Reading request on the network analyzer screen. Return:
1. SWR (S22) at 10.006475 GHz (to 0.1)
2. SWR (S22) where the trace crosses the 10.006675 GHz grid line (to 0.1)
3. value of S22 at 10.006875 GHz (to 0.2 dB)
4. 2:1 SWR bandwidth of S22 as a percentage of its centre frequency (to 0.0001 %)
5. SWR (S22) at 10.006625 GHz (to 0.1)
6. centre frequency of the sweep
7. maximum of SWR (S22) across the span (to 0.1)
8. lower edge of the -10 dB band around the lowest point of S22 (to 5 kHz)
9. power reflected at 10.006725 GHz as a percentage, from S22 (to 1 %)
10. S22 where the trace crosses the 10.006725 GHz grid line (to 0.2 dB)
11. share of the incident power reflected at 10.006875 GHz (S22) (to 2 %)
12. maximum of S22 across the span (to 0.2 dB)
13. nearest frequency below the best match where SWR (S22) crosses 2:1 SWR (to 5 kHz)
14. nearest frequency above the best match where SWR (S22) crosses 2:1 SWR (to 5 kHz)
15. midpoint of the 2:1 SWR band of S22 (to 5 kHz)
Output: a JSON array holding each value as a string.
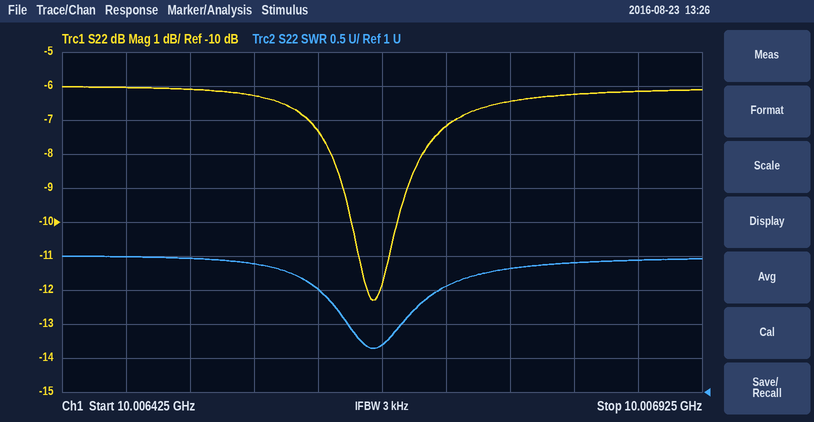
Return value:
["3.0", "1.7", "-6.2 dB", "0.0004 %", "2.5", "10.006675 GHz", "3.0", "10.006650 GHz", "19 %", "-7.2 dB", "24 %", "-6.0 dB", "10.006650 GHz", "10.006690 GHz", "10.006670 GHz"]
